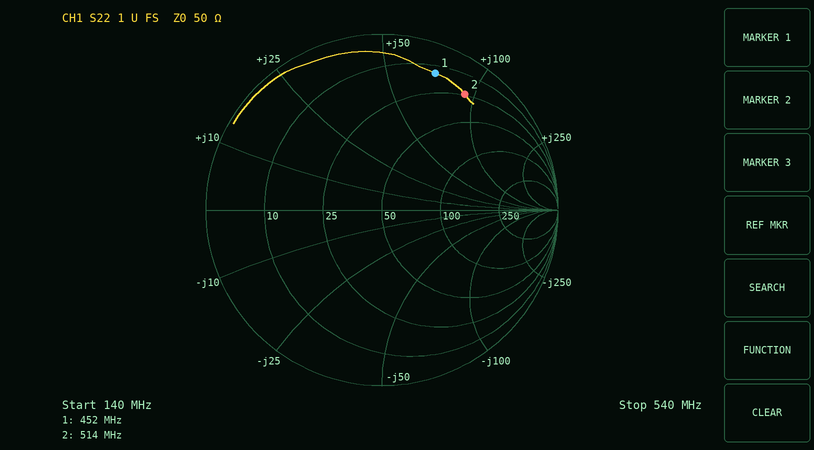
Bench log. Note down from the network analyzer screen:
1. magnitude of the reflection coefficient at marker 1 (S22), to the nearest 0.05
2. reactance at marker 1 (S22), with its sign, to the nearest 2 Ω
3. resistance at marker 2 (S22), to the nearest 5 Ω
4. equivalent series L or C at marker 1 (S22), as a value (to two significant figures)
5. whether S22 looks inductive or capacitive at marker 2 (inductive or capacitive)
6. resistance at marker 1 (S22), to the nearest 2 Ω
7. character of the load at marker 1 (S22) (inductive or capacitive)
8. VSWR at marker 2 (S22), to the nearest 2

0.85
+72 Ω
25 Ω
25 nH
inductive
14 Ω
inductive
10
